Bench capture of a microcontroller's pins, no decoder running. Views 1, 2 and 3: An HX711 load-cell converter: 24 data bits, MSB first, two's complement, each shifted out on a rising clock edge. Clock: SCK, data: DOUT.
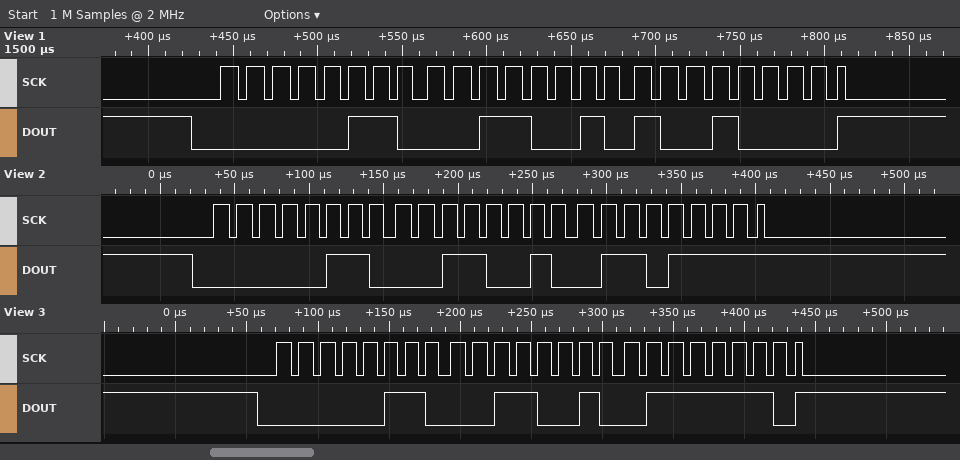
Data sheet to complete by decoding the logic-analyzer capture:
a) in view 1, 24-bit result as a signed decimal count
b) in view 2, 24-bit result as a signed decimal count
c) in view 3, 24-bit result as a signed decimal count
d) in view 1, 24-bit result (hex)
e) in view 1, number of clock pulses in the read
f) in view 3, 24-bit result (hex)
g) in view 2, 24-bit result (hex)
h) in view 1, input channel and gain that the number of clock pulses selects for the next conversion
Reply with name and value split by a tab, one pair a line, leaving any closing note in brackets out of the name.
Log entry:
in view 1, 24-bit result as a signed decimal count	406160
in view 2, 24-bit result as a signed decimal count	406127
in view 3, 24-bit result as a signed decimal count	406142
in view 1, 24-bit result	0x063290
in view 1, number of clock pulses in the read	25
in view 3, 24-bit result	0x06327E
in view 2, 24-bit result	0x06326F
in view 1, input channel and gain that the number of clock pulses selects for the next conversion	channel A, gain 128
